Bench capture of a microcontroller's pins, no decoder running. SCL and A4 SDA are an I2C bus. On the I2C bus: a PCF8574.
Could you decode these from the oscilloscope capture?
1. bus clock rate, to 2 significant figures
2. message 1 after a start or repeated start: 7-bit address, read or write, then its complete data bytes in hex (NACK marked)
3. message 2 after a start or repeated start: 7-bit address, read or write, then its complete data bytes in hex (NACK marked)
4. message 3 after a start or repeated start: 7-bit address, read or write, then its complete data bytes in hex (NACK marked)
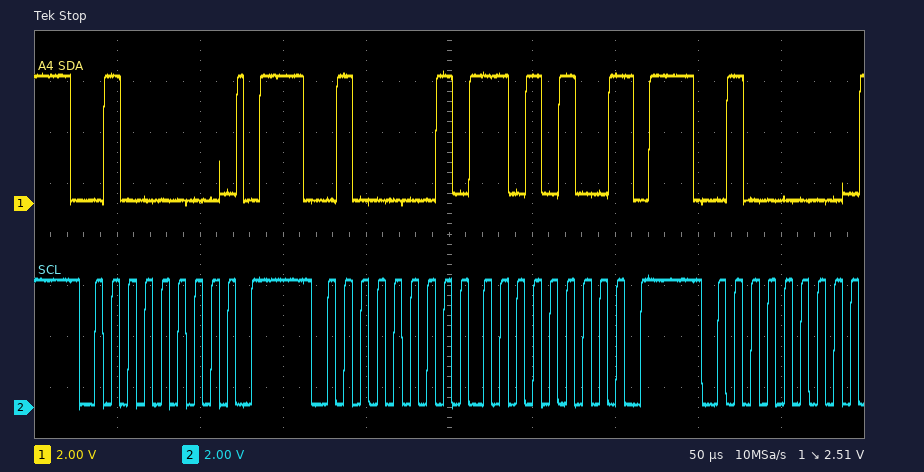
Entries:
100 kHz
0x20 write
0x20 read: D4 NACK
0x20 write
